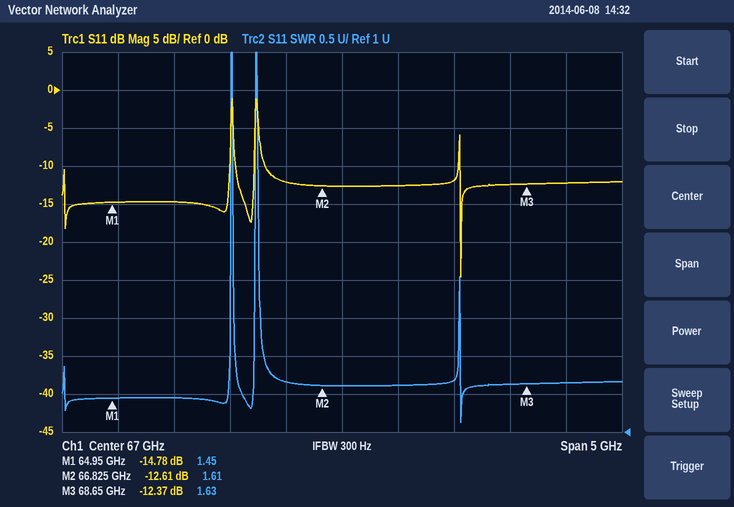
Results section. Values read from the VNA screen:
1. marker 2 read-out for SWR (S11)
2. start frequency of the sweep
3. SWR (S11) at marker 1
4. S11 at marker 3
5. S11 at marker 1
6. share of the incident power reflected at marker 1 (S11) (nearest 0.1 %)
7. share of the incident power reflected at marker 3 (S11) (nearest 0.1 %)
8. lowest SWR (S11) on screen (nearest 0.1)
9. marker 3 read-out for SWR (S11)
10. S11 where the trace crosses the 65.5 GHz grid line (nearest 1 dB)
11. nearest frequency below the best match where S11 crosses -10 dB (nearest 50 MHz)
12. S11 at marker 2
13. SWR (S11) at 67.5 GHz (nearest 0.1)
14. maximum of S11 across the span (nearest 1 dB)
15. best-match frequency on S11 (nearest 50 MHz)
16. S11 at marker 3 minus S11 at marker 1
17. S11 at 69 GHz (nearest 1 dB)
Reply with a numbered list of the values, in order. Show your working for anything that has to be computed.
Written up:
1. 1.61
2. 64.5 GHz
3. 1.45
4. -12.37 dB
5. -14.78 dB
6. 10^(-14.78/10) ≈ 3.3 %
7. 10^(-12.37/10) ≈ 5.8 %
8. 1.1
9. 1.63
10. -15 dB
11. 68.05 GHz
12. -12.61 dB
13. 1.6
14. -1 dB
15. 68.05 GHz
16. -12.37 − (-14.78) = 2.41 dB
17. -12 dB
